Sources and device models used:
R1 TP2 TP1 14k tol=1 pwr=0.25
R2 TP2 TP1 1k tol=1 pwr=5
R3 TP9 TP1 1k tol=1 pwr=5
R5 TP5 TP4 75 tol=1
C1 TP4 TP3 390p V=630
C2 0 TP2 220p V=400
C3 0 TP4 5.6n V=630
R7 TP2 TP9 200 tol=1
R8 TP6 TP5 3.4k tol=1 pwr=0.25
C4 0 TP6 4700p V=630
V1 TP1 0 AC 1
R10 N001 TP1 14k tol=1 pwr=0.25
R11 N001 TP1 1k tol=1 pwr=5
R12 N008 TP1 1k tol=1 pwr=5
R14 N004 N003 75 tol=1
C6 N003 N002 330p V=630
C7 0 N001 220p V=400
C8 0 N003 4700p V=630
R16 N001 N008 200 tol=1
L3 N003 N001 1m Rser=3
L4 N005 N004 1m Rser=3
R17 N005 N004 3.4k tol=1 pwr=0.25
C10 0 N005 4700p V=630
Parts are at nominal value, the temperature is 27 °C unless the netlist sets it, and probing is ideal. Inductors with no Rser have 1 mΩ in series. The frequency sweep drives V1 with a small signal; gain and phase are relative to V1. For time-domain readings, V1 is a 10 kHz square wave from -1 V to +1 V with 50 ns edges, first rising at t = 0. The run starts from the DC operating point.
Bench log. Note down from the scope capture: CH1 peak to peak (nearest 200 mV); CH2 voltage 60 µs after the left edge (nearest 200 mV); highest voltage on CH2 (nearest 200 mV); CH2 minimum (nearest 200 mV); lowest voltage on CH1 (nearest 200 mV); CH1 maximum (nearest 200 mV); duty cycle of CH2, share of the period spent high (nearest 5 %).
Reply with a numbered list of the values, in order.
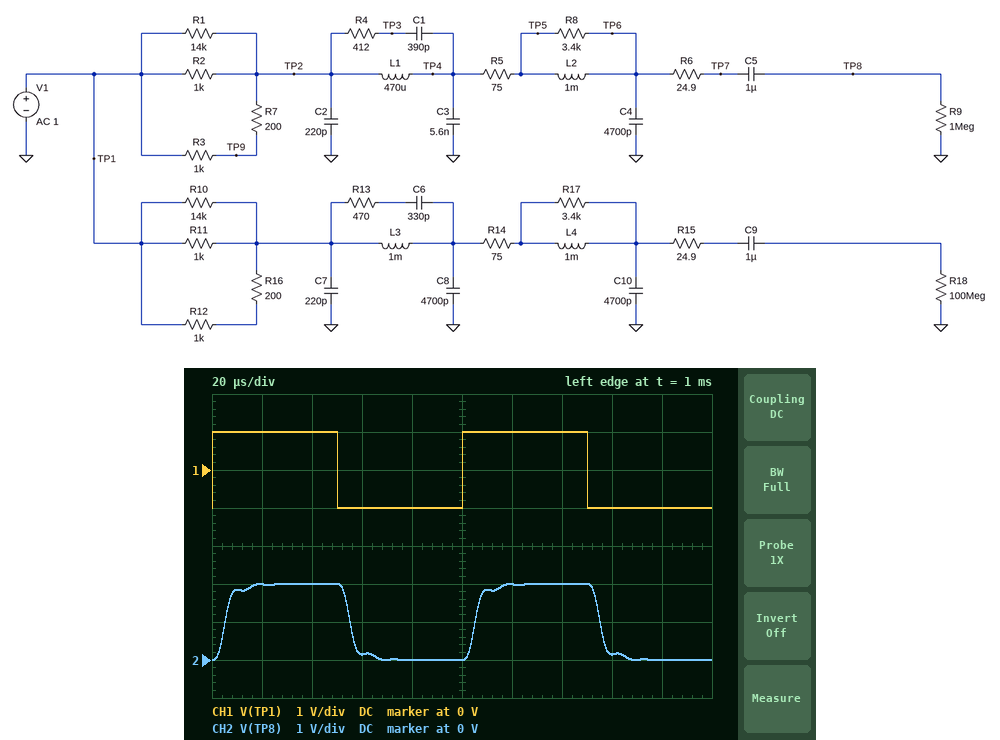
1. 2.0 V
2. 200 mV
3. 2.0 V
4. 0 V
5. -1.0 V
6. 1.0 V
7. 50 %
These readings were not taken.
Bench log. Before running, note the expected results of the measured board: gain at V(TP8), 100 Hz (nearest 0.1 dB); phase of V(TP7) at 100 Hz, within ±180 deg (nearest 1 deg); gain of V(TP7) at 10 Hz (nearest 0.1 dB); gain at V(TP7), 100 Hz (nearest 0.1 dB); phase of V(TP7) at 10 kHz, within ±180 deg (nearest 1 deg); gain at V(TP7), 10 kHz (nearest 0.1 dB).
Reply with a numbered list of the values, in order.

1. 0 dB
2. 0 deg
3. 0 dB
4. 0 dB
5. -21 deg
6. -0.2 dB
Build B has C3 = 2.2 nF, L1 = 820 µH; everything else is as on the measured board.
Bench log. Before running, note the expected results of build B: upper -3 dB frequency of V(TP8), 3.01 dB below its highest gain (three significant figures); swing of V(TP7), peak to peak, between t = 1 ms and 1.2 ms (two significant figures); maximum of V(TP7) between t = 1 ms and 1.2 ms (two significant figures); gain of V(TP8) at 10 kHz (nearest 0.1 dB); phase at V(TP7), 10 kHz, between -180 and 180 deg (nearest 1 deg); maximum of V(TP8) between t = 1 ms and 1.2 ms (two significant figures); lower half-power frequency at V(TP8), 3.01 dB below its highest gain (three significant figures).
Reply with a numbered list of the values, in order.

1. 63.0 kHz
2. 2.4 V
3. 1.2 V
4. 0.1 dB
5. -15 deg
6. 2.2 V
7. 173 mHz
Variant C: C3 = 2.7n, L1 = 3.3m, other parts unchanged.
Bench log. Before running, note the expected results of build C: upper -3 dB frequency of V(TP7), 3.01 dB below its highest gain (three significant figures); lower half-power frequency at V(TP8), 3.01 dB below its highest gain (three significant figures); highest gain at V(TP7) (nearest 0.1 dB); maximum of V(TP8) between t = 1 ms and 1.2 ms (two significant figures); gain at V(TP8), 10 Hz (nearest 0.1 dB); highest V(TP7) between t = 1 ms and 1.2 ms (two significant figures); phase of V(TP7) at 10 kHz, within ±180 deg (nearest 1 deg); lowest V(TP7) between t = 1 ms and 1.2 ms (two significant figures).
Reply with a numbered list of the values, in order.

1. 36.1 kHz
2. 5.03 kHz
3. 3.2 dB
4. 2.6 V
5. 0 dB
6. 1.6 V
7. -17 deg
8. -1.6 V
